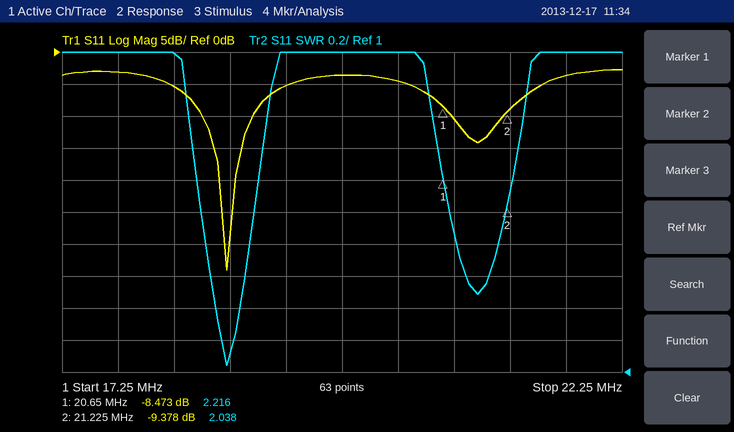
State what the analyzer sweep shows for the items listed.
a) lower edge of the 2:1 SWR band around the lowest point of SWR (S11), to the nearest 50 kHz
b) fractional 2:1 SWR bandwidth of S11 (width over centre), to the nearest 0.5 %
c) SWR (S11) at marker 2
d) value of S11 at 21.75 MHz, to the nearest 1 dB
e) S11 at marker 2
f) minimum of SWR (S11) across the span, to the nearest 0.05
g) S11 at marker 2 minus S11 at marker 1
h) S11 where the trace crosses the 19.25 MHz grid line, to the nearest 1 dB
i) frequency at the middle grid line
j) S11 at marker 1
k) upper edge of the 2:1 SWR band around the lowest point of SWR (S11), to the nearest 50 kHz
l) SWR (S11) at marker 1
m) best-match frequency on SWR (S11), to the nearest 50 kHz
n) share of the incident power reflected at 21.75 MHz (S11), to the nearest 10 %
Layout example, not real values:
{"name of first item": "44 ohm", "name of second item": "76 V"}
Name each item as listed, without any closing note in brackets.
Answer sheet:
{"lower edge of the 2:1 SWR band around the lowest point of SWR (S11), to the nearest 50 kHz": "18.50 MHz", "fractional 2:1 SWR bandwidth of S11 (width over centre), to the nearest 0.5 %": "2.5 %", "SWR (S11) at marker 2": "2.038", "value of S11 at 21.75 MHz, to the nearest 1 dB": "-4 dB", "S11 at marker 2": "-9.378 dB", "minimum of SWR (S11) across the span, to the nearest 0.05": "1.05", "S11 at marker 2 minus S11 at marker 1": "-0.905 dB", "S11 where the trace crosses the 19.25 MHz grid line, to the nearest 1 dB": "-5 dB", "frequency at the middle grid line": "19.75 MHz", "S11 at marker 1": "-8.473 dB", "upper edge of the 2:1 SWR band around the lowest point of SWR (S11), to the nearest 50 kHz": "18.95 MHz", "SWR (S11) at marker 1": "2.216", "best-match frequency on SWR (S11), to the nearest 50 kHz": "18.70 MHz", "share of the incident power reflected at 21.75 MHz (S11), to the nearest 10 %": "40 %"}
